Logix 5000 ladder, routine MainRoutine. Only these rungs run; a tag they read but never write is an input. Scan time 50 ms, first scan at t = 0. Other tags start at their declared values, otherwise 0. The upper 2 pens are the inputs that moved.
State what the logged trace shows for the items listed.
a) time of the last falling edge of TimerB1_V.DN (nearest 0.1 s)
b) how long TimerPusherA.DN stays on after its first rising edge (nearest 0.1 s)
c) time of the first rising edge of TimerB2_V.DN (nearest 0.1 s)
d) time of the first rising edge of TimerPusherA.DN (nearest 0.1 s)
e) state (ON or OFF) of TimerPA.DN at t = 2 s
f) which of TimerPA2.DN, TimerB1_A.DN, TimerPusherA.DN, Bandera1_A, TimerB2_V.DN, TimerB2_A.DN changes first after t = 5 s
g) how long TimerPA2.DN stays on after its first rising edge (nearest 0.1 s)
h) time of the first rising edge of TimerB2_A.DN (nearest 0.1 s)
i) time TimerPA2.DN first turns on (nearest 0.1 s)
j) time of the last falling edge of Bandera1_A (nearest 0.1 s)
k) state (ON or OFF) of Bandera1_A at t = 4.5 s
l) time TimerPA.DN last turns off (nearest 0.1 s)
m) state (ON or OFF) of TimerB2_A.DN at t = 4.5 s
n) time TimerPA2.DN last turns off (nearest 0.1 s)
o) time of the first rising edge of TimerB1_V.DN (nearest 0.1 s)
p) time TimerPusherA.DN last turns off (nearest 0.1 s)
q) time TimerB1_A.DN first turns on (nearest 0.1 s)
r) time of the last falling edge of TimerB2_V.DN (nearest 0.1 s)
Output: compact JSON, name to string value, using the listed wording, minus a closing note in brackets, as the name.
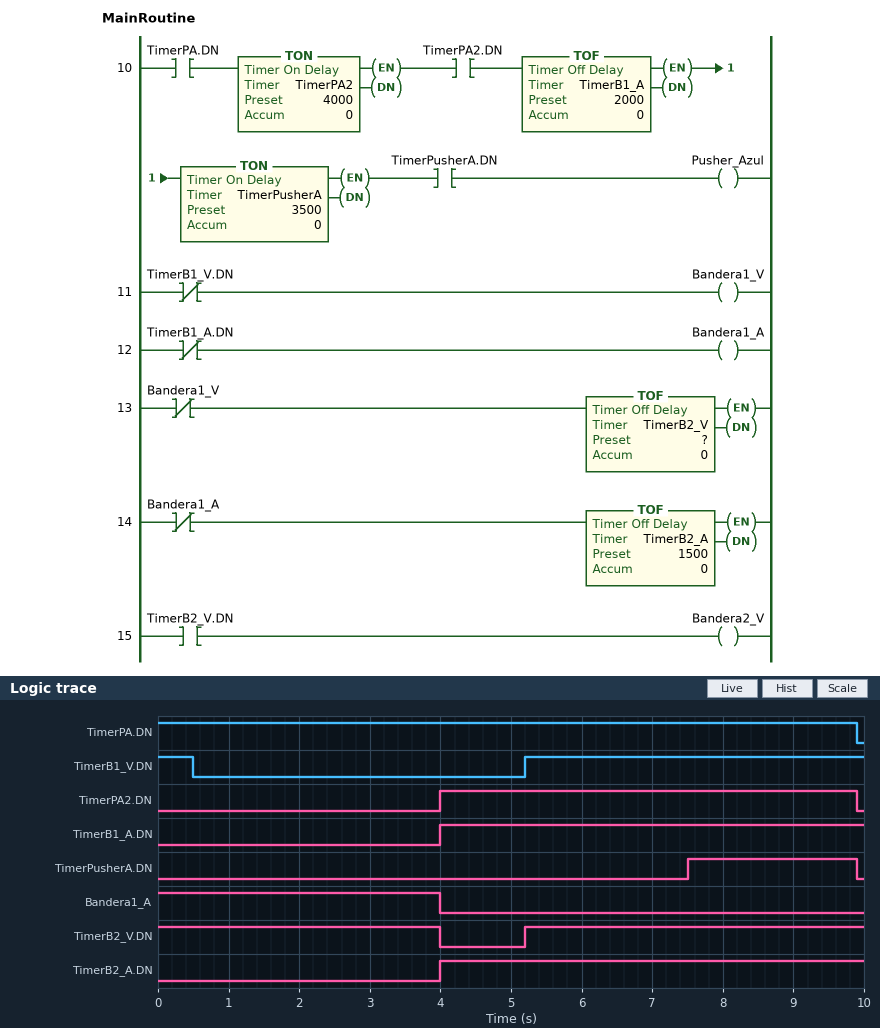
{"time of the last falling edge of TimerB1_V.DN": "0.5 s", "how long TimerPusherA.DN stays on after its first rising edge": "2.4 s", "time of the first rising edge of TimerB2_V.DN": "5.2 s", "time of the first rising edge of TimerPusherA.DN": "7.5 s", "state (ON or OFF) of TimerPA.DN at t = 2 s": "ON", "which of TimerPA2.DN, TimerB1_A.DN, TimerPusherA.DN, Bandera1_A, TimerB2_V.DN, TimerB2_A.DN changes first after t = 5 s": "TimerB2_V.DN", "how long TimerPA2.DN stays on after its first rising edge": "5.9 s", "time of the first rising edge of TimerB2_A.DN": "4.0 s", "time TimerPA2.DN first turns on": "4.0 s", "time of the last falling edge of Bandera1_A": "4.0 s", "state (ON or OFF) of Bandera1_A at t = 4.5 s": "OFF", "time TimerPA.DN last turns off": "9.9 s", "state (ON or OFF) of TimerB2_A.DN at t = 4.5 s": "ON", "time TimerPA2.DN last turns off": "9.9 s", "time of the first rising edge of TimerB1_V.DN": "5.2 s", "time TimerPusherA.DN last turns off": "9.9 s", "time TimerB1_A.DN first turns on": "4.0 s", "time of the last falling edge of TimerB2_V.DN": "4.0 s"}
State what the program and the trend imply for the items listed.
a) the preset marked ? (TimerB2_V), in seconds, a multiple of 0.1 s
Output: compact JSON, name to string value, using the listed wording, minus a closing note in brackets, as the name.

{"the preset marked ? (TimerB2_V), in seconds, a multiple of 0.1 s": "3.5 s"}
